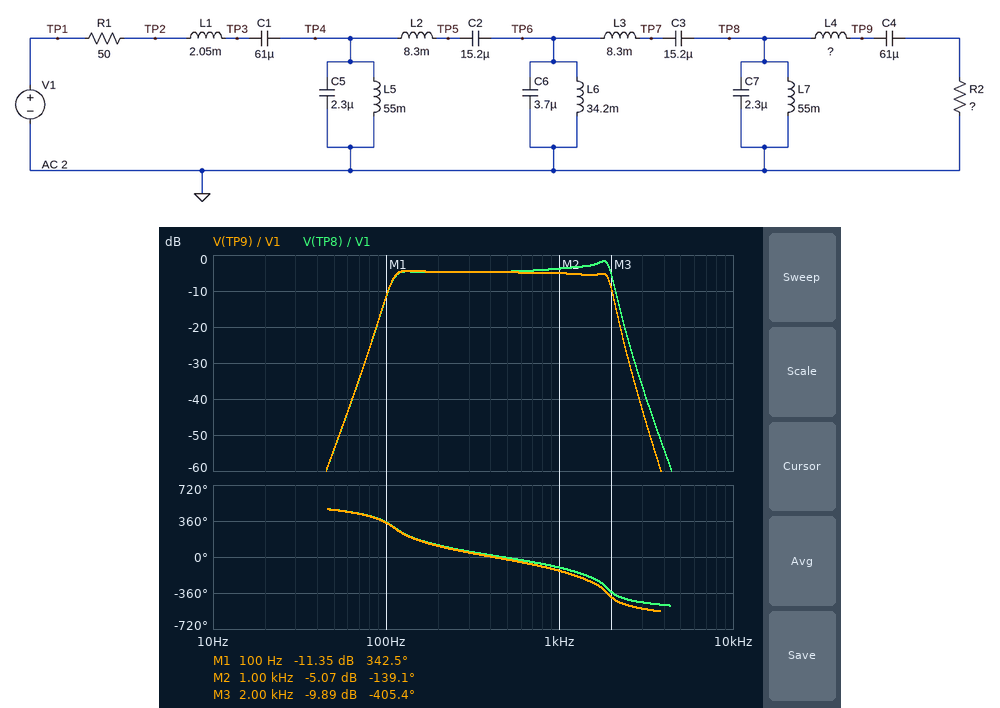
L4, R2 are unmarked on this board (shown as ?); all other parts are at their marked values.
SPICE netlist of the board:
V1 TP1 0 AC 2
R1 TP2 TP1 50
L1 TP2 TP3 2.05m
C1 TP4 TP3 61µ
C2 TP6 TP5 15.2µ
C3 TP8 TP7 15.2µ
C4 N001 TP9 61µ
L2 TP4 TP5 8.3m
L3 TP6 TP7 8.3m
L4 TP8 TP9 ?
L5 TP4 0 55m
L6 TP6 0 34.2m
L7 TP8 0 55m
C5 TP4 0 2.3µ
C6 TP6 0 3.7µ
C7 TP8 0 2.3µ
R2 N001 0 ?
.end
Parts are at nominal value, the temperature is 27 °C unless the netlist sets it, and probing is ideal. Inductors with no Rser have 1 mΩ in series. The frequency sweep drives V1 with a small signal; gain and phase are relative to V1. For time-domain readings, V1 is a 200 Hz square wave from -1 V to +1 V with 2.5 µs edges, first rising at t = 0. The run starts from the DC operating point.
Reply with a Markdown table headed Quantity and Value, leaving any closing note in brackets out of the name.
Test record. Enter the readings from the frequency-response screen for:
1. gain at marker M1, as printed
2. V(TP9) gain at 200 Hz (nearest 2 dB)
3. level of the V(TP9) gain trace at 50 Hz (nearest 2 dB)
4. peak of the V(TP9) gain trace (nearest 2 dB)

| Quantity | Value |
|---|---|
| gain at marker M1, as printed | -11.35 dB |
| V(TP9) gain at 200 Hz | -4 dB |
| level of the V(TP9) gain trace at 50 Hz | -54 dB |
| peak of the V(TP9) gain trace | -4 dB |
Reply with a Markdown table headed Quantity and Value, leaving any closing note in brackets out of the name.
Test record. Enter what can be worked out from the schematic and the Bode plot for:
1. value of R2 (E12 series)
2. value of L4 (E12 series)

| Quantity | Value |
|---|---|
| value of R2 | 68 Ω |
| value of L4 | 6.8 mH |
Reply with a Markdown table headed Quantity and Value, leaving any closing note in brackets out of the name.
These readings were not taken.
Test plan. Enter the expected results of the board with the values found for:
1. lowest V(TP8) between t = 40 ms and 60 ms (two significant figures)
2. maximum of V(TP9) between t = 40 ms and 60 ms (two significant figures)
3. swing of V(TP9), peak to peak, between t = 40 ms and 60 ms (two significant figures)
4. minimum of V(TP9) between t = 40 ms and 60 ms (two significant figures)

| Quantity | Value |
|---|---|
| lowest V(TP8) between t = 40 ms and 60 ms | -980 mV |
| maximum of V(TP9) between t = 40 ms and 60 ms | 890 mV |
| swing of V(TP9), peak to peak, between t = 40 ms and 60 ms | 1.8 V |
| minimum of V(TP9) between t = 40 ms and 60 ms | -890 mV |
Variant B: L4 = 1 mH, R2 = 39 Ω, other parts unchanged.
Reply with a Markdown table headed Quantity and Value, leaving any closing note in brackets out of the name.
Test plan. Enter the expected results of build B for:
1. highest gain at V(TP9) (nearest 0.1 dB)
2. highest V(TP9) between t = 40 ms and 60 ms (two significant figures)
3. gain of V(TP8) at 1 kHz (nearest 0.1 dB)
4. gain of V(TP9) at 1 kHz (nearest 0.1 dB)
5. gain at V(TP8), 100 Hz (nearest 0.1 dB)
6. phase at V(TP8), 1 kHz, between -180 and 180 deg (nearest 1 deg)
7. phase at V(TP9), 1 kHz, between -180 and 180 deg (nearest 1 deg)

| Quantity | Value |
|---|---|
| highest gain at V(TP9) | -6.4 dB |
| highest V(TP9) between t = 40 ms and 60 ms | 750 mV |
| gain of V(TP8) at 1 kHz | -7.1 dB |
| gain of V(TP9) at 1 kHz | -7.2 dB |
| gain at V(TP8), 100 Hz | -12.6 dB |
| phase at V(TP8), 1 kHz, between -180 and 180 deg | -113 deg |
| phase at V(TP9), 1 kHz, between -180 and 180 deg | -122 deg |
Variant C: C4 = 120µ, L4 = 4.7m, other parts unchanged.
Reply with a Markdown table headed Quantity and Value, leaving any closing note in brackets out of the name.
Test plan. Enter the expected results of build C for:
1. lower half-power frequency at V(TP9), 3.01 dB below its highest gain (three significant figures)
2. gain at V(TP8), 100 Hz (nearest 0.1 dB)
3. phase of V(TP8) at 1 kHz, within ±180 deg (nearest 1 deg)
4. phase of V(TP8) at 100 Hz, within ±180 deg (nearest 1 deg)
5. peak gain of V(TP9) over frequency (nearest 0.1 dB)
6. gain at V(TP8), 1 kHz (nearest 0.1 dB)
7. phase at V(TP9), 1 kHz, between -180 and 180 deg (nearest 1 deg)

| Quantity | Value |
|---|---|
| lower half-power frequency at V(TP9), 3.01 dB below its highest gain | 109 Hz |
| gain at V(TP8), 100 Hz | -12.5 dB |
| phase of V(TP8) at 1 kHz, within ±180 deg | -109 deg |
| phase of V(TP8) at 100 Hz, within ±180 deg | -10 deg |
| peak gain of V(TP9) over frequency | -4.6 dB |
| gain at V(TP8), 1 kHz | -4.2 dB |
| phase at V(TP9), 1 kHz, between -180 and 180 deg | -132 deg |
